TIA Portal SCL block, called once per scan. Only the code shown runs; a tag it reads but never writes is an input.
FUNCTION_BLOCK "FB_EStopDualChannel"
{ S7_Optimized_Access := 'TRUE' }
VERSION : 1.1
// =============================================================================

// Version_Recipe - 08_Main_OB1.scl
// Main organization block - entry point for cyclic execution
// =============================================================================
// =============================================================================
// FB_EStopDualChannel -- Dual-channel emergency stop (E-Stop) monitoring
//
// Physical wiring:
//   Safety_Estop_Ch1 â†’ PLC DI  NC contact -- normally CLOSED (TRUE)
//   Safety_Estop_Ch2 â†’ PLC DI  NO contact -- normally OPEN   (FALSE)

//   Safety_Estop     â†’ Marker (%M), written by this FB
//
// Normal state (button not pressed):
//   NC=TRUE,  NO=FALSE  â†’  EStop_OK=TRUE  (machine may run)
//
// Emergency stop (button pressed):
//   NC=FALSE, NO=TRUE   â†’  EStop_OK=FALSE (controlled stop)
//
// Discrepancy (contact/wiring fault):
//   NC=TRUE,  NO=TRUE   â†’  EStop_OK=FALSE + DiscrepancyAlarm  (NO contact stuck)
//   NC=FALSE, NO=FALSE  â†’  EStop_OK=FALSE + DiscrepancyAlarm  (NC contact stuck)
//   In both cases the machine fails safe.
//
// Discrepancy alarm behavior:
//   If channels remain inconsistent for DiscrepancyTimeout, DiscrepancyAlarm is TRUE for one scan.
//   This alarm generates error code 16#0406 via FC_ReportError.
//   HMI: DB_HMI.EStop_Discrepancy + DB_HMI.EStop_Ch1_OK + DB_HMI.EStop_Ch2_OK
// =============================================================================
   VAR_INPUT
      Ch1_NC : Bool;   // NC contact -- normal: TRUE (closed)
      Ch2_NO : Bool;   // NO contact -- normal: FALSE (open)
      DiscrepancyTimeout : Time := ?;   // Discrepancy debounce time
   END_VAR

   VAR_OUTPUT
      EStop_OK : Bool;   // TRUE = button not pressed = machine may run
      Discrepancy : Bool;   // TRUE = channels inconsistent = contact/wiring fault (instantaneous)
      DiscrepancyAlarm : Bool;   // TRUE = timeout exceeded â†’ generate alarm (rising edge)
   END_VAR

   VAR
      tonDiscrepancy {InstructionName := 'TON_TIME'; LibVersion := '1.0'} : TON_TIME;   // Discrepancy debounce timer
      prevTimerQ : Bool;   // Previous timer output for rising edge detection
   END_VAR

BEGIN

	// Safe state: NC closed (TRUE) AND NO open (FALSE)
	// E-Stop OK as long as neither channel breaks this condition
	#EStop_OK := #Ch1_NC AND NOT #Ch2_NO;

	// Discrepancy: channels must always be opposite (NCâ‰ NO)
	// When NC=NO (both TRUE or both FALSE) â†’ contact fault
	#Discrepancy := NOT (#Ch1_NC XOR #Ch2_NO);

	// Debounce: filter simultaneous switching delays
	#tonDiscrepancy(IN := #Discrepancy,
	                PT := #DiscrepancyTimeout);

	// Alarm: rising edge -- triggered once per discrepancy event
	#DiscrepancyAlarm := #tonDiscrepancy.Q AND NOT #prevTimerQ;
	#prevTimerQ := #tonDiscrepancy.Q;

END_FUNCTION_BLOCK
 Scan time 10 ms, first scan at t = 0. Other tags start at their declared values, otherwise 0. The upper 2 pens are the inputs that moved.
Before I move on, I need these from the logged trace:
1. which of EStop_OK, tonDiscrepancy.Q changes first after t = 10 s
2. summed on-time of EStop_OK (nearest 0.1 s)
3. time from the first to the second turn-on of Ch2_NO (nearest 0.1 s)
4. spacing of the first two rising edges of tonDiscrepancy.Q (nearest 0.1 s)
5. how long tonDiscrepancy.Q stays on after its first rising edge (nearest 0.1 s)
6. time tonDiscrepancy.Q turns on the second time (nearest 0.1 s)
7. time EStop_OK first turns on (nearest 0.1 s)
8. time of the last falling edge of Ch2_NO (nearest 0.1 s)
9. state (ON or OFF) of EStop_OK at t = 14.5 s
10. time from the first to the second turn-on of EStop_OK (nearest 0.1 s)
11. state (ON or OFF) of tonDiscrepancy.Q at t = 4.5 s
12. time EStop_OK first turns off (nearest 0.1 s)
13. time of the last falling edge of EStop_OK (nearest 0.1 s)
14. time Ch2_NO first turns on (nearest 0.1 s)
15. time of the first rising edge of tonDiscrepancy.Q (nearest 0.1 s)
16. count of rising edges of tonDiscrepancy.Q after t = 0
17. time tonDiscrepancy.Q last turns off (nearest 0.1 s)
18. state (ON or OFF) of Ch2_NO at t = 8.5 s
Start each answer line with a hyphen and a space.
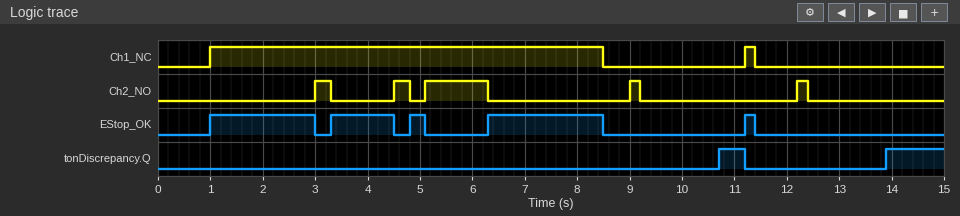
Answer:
- tonDiscrepancy.Q
- 5.9 s
- 1.5 s
- 3.2 s
- 0.5 s
- 13.9 s
- 1.0 s
- 12.4 s
- OFF
- 2.3 s
- OFF
- 3.0 s
- 11.4 s
- 3.0 s
- 10.7 s
- 2
- 11.2 s
- OFF
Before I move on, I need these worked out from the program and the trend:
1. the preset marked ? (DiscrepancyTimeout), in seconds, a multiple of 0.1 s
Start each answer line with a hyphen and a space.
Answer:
- 1.5 s
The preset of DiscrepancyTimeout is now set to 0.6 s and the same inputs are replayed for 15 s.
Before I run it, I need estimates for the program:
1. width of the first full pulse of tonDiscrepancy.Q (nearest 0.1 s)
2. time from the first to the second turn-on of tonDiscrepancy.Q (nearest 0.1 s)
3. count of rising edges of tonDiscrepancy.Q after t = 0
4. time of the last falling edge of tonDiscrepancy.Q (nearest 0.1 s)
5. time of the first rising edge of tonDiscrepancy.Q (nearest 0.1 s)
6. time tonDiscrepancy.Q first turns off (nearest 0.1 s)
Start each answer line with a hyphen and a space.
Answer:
- 0.4 s
- 5.1 s
- 5
- 12.2 s
- 0.6 s
- 1.0 s
